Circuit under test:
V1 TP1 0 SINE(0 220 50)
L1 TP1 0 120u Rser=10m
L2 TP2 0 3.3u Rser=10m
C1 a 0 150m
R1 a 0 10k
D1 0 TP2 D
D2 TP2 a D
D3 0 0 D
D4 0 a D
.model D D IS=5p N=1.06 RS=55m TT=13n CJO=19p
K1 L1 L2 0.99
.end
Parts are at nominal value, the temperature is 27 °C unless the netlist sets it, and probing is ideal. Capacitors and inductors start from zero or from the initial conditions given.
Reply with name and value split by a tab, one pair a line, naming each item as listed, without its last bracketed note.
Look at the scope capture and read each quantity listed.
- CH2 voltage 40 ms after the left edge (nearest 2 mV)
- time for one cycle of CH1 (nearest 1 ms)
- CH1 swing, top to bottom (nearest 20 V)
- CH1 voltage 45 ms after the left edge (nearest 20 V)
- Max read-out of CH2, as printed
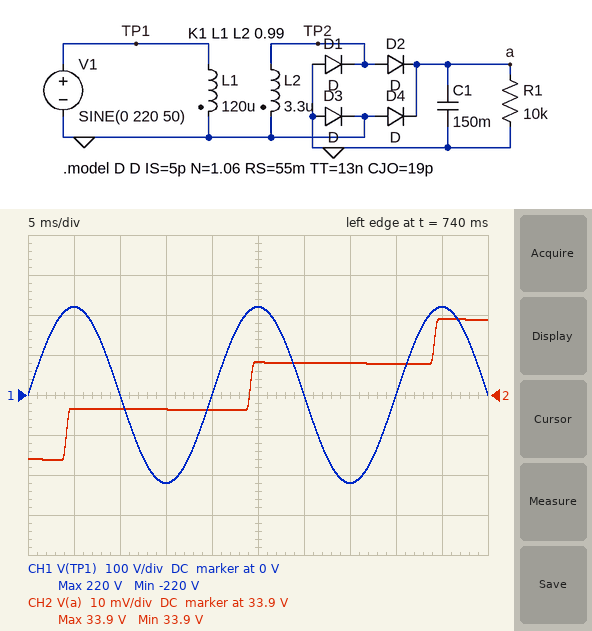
CH2 voltage 40 ms after the left edge	33.908 V
time for one cycle of CH1	20 ms
CH1 swing, top to bottom	440 V
CH1 voltage 45 ms after the left edge	220 V
Max read-out of CH2, as printed	33.9 V
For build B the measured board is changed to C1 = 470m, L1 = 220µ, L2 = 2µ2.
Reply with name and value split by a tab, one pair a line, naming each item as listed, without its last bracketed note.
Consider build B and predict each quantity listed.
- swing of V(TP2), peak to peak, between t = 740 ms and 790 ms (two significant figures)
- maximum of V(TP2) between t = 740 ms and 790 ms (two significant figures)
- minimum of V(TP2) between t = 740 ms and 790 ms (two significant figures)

swing of V(TP2), peak to peak, between t = 740 ms and 790 ms	40 V
maximum of V(TP2) between t = 740 ms and 790 ms	21 V
minimum of V(TP2) between t = 740 ms and 790 ms	-18 V
